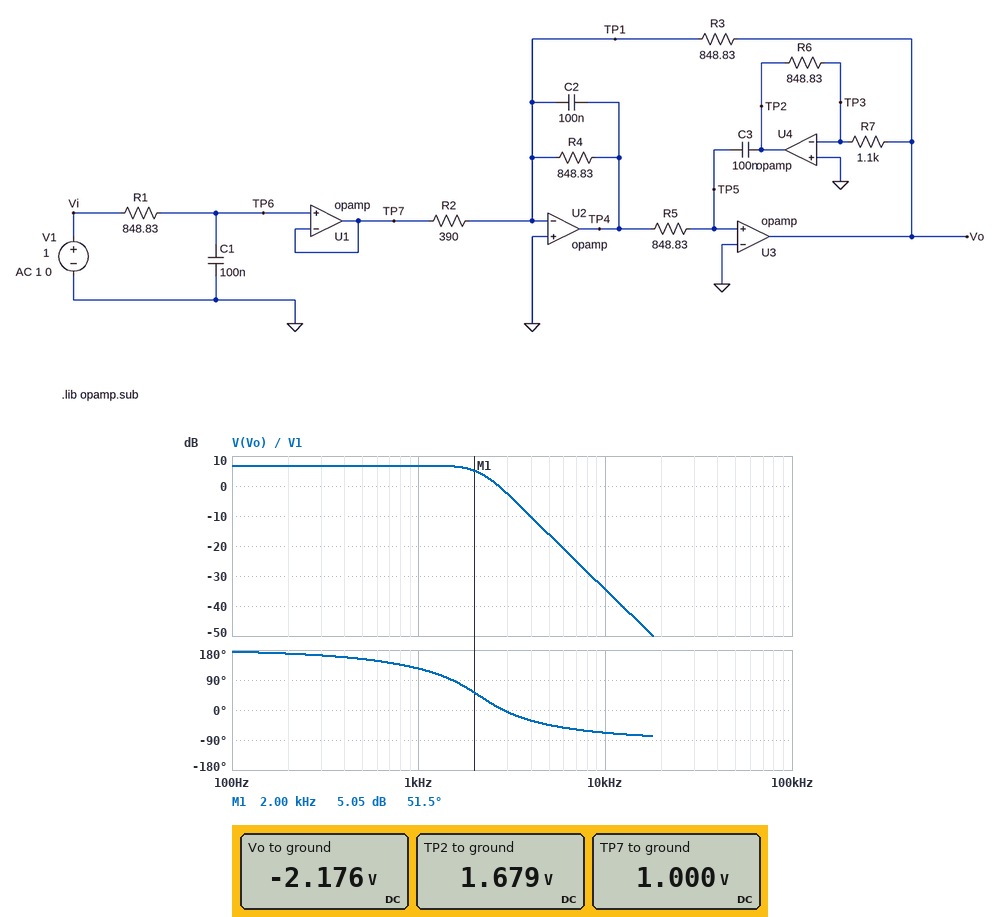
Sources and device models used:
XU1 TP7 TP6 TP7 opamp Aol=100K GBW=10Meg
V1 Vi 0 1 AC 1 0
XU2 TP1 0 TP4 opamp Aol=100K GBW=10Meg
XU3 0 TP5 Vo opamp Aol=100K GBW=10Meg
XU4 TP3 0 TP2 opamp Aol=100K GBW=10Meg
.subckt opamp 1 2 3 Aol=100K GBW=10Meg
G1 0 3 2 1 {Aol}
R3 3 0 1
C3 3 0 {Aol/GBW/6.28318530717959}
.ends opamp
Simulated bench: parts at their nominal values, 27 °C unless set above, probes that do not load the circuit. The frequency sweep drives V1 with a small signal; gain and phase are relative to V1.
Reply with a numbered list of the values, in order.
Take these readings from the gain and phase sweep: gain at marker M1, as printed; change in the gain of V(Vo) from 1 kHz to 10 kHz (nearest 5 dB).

1. 5.05 dB
2. -40 dB
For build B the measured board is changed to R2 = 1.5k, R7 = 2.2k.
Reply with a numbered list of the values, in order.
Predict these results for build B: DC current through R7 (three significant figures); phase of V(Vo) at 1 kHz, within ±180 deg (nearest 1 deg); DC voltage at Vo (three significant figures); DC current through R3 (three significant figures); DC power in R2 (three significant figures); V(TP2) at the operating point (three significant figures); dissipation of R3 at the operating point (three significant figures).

1. 257 µA
2. 139 deg
3. -566 mV
4. 667 µA
5. 667 µW
6. 218 mV
7. 377 µW
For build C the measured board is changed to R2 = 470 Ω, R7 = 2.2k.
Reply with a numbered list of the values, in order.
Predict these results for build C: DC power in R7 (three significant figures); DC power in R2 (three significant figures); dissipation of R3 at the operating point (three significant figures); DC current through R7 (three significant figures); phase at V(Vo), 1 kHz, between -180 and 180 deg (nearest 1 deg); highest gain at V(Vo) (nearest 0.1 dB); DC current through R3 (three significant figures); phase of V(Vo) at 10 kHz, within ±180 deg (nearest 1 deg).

1. 1.48 mW
2. 2.13 mW
3. 3.84 mW
4. 821 µA
5. 139 deg
6. 5.1 dB
7. 2.13 mA
8. -68 deg
